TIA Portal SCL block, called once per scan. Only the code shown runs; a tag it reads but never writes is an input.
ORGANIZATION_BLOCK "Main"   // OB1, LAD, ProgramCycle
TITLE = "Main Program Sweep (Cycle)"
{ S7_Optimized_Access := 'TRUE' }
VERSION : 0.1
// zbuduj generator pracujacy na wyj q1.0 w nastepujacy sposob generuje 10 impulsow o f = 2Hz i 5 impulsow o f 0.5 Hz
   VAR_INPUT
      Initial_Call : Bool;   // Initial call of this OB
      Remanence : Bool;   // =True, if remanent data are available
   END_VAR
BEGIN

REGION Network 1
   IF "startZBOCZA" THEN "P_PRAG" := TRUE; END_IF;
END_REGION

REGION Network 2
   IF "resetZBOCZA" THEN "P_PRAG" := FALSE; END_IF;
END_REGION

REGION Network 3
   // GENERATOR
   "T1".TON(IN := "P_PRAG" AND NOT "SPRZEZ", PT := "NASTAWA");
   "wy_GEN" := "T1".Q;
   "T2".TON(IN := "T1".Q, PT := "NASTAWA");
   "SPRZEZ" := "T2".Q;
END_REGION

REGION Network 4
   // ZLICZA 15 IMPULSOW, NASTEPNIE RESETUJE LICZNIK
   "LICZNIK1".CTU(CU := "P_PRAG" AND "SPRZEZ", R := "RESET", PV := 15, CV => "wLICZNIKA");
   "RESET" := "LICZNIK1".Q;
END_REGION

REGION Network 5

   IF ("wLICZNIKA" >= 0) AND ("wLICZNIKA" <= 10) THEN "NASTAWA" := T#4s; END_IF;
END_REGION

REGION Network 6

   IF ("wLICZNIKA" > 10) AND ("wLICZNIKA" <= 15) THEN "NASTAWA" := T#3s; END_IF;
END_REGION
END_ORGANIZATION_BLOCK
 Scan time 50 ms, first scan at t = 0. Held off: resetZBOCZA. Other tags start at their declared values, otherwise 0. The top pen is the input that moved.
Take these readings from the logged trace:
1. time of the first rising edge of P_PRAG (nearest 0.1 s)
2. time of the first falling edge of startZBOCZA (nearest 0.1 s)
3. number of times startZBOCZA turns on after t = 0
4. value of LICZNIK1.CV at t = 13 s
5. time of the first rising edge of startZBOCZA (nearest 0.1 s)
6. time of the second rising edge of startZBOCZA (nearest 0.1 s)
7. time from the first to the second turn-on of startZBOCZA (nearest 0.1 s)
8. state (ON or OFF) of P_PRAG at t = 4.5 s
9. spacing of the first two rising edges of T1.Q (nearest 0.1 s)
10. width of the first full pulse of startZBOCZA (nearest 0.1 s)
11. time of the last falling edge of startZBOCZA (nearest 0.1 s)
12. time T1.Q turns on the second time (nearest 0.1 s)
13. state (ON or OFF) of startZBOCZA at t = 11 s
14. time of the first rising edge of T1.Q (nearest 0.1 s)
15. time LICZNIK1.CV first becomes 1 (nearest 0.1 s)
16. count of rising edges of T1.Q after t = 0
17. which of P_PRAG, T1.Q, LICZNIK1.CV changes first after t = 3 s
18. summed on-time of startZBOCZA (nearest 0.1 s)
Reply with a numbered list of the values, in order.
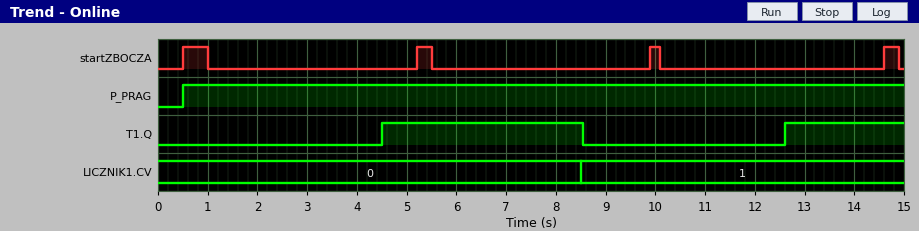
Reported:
1. 0.5 s
2. 1.0 s
3. 4
4. 1
5. 0.5 s
6. 5.2 s
7. 4.7 s
8. ON
9. 8.1 s
10. 0.5 s
11. 14.9 s
12. 12.6 s
13. OFF
14. 4.5 s
15. 8.5 s
16. 2
17. T1.Q
18. 1.3 s
